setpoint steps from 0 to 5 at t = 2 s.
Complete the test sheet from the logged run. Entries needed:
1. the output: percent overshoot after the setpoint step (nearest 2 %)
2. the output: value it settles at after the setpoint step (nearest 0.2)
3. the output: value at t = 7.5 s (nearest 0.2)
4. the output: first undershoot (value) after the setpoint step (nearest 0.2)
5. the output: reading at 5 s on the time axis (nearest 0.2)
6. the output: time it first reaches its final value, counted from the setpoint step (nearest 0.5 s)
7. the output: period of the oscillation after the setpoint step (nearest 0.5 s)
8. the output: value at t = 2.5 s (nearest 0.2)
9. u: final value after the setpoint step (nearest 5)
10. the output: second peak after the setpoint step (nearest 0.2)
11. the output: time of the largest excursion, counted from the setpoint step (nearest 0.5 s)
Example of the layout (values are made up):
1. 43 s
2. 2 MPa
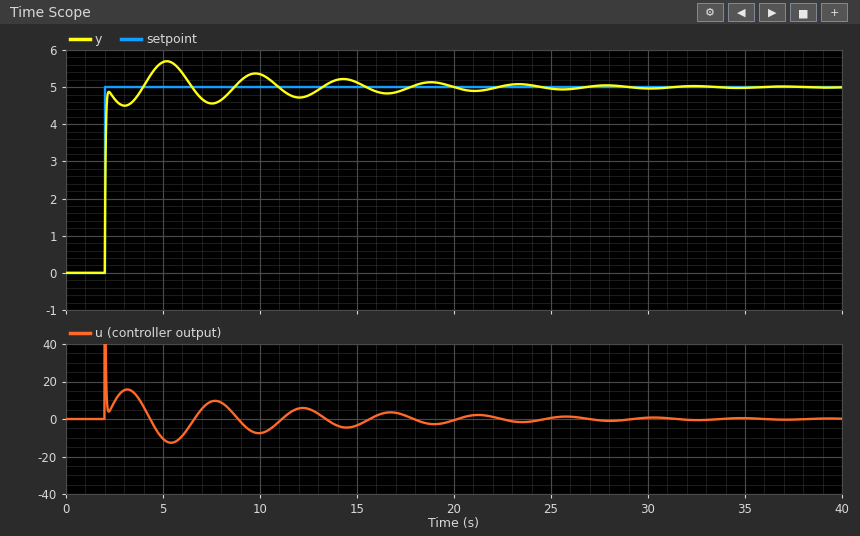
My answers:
1. 14 %
2. 5.0
3. 4.6
4. 4.6
5. 5.6
6. 2.0 s
7. 4.5 s
8. 4.6
9. 0
10. 5.4
11. 3.0 s
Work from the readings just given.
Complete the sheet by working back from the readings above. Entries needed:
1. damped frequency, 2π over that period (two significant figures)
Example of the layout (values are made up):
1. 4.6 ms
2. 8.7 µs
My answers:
1. 1.4 rad/s
